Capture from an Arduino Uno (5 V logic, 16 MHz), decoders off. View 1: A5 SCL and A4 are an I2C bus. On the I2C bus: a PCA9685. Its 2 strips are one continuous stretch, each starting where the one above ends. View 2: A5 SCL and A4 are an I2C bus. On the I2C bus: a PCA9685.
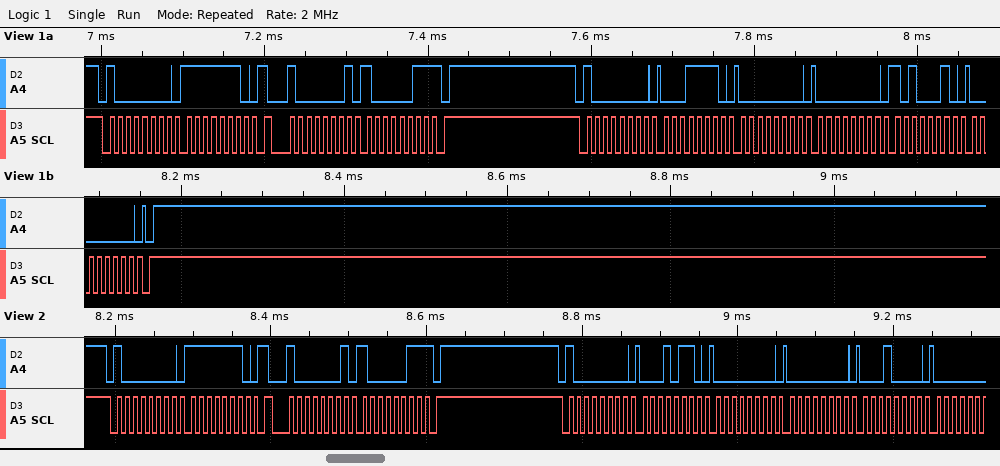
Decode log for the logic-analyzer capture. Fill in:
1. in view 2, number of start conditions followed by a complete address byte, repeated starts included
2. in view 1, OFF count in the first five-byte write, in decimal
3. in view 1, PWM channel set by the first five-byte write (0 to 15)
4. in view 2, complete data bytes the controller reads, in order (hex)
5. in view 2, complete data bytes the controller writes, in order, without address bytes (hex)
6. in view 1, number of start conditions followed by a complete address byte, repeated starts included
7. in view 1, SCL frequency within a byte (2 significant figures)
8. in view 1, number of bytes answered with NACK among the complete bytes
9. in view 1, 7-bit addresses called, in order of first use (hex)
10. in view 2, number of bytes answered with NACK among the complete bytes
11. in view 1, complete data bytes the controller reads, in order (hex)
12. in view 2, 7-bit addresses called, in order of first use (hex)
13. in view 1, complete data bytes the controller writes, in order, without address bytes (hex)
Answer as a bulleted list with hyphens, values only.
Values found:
- 3
- 162
- 6
- 83
- FE 16 00 00 10
- 3
- 100 kHz
- 1
- 0x40
- 1
- 83
- 0x40
- FE 1E 00 00 A2 00
